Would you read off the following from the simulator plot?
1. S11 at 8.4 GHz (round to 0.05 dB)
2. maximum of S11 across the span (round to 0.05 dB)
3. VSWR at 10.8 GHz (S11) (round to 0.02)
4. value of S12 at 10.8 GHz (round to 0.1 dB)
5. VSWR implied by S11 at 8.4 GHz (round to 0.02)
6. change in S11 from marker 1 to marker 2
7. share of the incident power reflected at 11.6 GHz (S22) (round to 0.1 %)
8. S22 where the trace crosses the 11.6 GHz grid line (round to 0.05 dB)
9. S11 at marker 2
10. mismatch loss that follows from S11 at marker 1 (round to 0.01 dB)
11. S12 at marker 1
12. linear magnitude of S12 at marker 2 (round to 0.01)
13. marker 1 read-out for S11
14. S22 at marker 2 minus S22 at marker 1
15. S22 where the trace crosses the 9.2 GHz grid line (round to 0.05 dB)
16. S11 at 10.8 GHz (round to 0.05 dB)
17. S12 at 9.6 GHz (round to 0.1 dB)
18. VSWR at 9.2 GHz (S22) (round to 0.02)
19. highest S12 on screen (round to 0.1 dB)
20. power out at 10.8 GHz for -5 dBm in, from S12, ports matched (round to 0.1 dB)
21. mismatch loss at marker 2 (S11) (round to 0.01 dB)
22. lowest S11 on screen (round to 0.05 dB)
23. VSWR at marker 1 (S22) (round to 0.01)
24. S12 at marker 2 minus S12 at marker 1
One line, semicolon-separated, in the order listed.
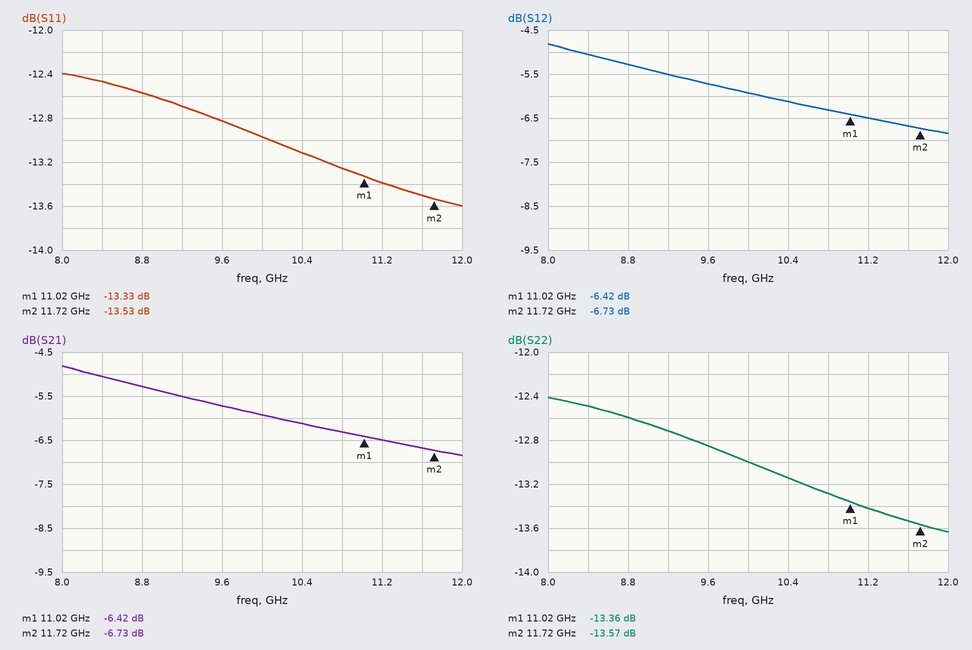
-12.45 dB; -12.40 dB; 1.56; -6.3 dB; 1.62; -0.20 dB; 4.4 %; -13.55 dB; -13.53 dB; 0.21 dB; -6.42 dB; 0.46; -13.33 dB; -0.21 dB; -12.70 dB; -13.25 dB; -5.7 dB; 1.60; -4.8 dB; -11.3 dBm; 0.20 dB; -13.60 dB; 1.55; -0.31 dB
